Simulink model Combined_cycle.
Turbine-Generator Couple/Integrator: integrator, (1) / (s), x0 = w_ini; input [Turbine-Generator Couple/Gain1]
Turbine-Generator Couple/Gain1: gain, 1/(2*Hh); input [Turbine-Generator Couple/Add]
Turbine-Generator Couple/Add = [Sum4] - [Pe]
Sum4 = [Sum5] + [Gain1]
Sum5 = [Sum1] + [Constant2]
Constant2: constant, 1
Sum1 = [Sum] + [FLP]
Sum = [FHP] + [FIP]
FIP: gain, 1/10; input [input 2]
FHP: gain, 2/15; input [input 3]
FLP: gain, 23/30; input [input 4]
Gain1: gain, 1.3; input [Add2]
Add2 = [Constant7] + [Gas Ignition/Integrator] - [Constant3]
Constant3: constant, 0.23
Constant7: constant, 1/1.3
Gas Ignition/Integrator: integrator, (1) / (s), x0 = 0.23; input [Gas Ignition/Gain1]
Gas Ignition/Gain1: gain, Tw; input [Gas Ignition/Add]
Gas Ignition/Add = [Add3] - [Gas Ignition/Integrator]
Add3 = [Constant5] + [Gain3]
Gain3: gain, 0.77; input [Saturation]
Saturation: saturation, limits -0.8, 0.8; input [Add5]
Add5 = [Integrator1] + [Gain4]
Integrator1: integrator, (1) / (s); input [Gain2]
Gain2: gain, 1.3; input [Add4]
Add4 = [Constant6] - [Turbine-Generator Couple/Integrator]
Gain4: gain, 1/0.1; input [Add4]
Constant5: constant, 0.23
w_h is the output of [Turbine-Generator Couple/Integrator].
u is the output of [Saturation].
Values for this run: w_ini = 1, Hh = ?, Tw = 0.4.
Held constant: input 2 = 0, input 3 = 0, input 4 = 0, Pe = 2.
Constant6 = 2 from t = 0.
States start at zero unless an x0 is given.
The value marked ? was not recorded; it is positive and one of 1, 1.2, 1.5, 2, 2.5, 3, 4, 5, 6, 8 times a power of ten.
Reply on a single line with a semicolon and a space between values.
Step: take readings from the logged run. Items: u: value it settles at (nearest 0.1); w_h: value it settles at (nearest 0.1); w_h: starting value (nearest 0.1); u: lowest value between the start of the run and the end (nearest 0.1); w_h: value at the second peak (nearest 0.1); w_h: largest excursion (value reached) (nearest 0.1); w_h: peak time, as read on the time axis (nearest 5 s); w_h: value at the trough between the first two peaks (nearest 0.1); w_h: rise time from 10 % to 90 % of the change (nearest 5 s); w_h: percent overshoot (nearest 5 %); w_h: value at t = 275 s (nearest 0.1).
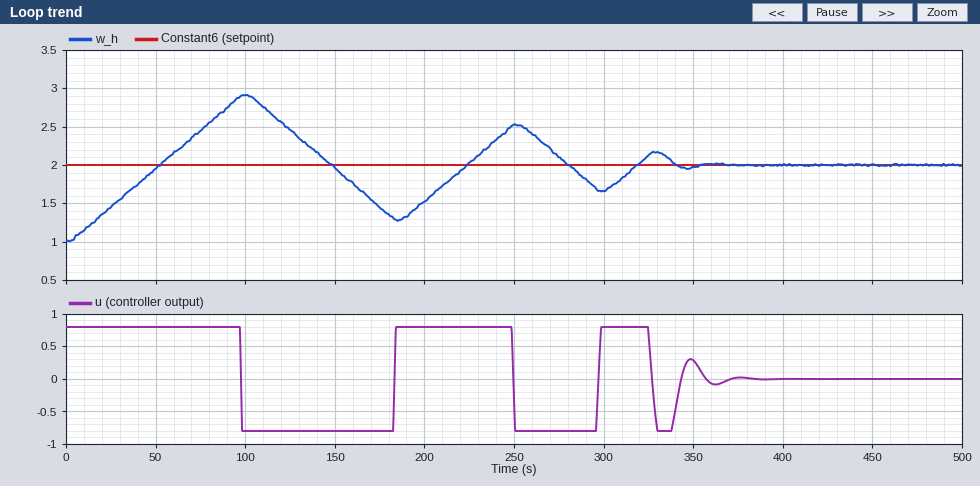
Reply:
0.0; 2.0; 1.0; -0.8; 2.5; 2.9; 100 s; 1.3; 40 s; 90 %; 2.1
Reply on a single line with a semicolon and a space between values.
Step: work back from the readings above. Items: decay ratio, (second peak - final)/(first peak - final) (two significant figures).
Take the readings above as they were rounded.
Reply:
0.56
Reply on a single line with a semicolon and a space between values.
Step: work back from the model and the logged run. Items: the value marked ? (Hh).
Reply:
20
